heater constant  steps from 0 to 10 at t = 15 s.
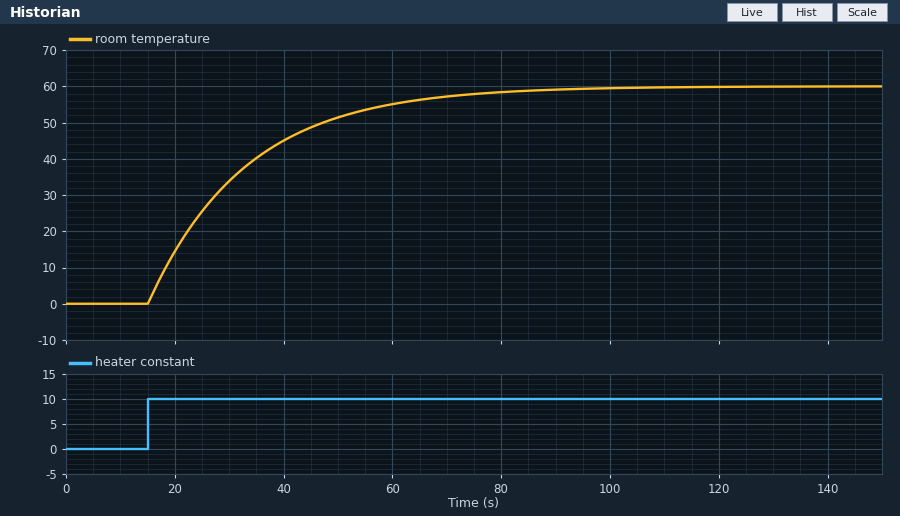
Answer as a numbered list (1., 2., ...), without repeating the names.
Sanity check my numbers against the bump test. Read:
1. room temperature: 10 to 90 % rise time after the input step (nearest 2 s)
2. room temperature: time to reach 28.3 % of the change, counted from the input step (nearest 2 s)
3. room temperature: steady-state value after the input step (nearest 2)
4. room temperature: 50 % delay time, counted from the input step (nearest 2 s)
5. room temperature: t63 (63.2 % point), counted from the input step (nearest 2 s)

1. 40 s
2. 6 s
3. 60
4. 12 s
5. 18 s
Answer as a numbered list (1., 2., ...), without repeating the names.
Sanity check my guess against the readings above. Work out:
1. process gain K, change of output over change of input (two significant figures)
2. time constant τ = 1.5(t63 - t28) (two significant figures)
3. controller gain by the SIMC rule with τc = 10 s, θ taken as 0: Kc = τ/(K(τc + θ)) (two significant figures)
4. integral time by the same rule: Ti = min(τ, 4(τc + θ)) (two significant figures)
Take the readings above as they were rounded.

1. 6.0
2. 18 s
3. 0.30
4. 18 s
